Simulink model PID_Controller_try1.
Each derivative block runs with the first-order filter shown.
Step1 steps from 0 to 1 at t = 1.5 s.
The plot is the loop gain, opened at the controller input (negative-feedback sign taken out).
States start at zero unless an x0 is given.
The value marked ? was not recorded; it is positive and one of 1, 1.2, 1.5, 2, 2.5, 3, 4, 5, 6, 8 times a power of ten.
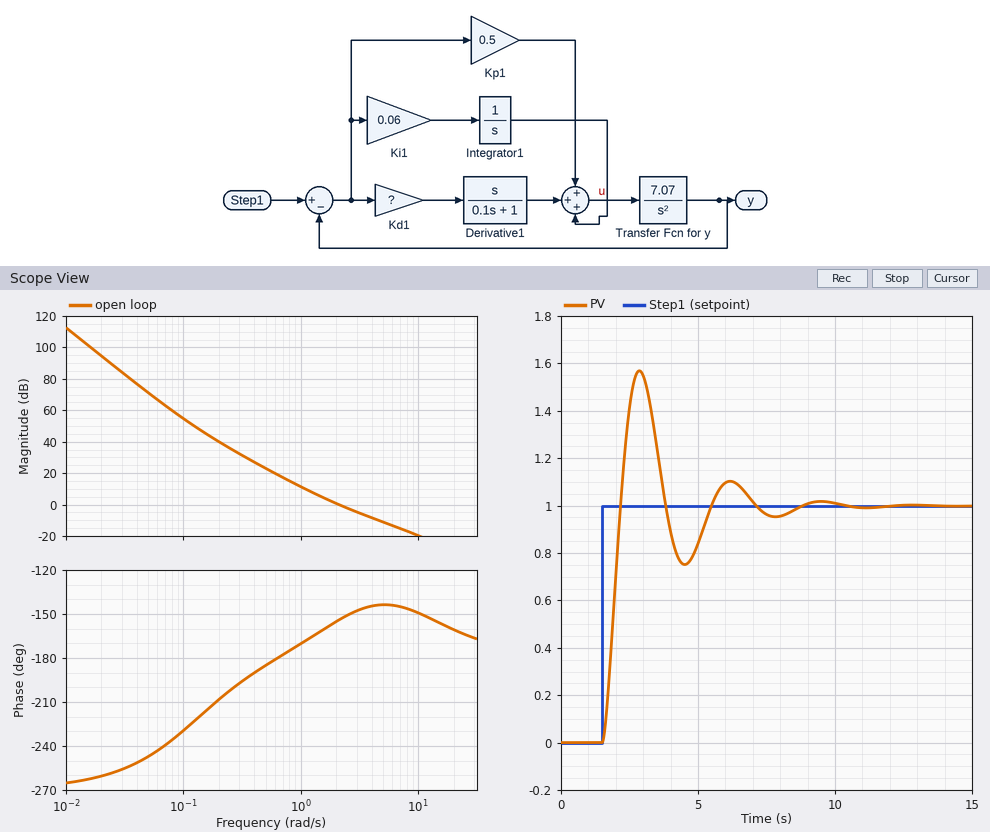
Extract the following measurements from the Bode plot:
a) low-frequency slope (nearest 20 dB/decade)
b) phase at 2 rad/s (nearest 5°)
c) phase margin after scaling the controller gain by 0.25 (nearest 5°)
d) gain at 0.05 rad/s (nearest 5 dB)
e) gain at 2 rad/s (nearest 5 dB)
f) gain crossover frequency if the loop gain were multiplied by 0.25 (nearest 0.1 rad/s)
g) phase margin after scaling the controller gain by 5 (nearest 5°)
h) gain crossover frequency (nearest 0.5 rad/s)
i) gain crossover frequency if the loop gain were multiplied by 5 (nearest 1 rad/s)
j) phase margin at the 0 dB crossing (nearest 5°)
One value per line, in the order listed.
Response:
-60 dB/decade
-155°
10°
70 dB
0 dB
1.0 rad/s
35°
2.0 rad/s
6 rad/s
25°
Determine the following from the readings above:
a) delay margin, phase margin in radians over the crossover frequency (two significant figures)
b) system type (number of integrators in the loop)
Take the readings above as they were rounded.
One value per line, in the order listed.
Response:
0.22 s
3
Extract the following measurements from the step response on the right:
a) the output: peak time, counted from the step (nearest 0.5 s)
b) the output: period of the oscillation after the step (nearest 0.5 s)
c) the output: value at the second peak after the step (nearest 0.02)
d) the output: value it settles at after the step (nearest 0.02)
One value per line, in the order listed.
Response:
1.5 s
3.5 s
1.10
1.00
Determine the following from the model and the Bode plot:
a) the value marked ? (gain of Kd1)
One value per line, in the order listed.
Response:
0.15
